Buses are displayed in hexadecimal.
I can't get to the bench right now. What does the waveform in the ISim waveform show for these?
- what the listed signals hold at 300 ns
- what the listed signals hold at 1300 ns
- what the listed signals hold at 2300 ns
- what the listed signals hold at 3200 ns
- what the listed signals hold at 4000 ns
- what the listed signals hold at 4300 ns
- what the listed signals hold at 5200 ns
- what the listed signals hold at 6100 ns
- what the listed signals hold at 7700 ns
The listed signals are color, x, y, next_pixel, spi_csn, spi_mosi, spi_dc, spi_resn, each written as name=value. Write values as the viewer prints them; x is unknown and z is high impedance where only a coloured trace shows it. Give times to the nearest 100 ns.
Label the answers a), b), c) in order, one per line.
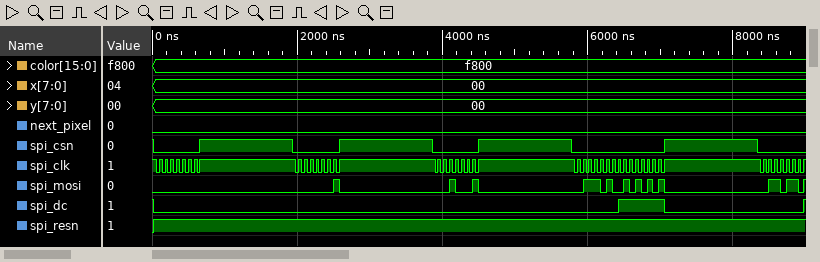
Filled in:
a) color=f800, x=00, y=00, next_pixel=0, spi_csn=0, spi_mosi=0, spi_dc=0, spi_resn=1
b) color=f800, x=00, y=00, next_pixel=0, spi_csn=1, spi_mosi=0, spi_dc=0, spi_resn=1
c) color=f800, x=00, y=00, next_pixel=0, spi_csn=0, spi_mosi=0, spi_dc=0, spi_resn=1
d) color=f800, x=00, y=00, next_pixel=0, spi_csn=1, spi_mosi=0, spi_dc=0, spi_resn=1
e) color=f800, x=00, y=00, next_pixel=0, spi_csn=0, spi_mosi=0, spi_dc=0, spi_resn=1
f) color=f800, x=00, y=00, next_pixel=0, spi_csn=0, spi_mosi=0, spi_dc=0, spi_resn=1
g) color=f800, x=00, y=00, next_pixel=0, spi_csn=1, spi_mosi=0, spi_dc=0, spi_resn=1
h) color=f800, x=00, y=00, next_pixel=0, spi_csn=0, spi_mosi=1, spi_dc=0, spi_resn=1
i) color=f800, x=00, y=00, next_pixel=0, spi_csn=1, spi_mosi=0, spi_dc=0, spi_resn=1
